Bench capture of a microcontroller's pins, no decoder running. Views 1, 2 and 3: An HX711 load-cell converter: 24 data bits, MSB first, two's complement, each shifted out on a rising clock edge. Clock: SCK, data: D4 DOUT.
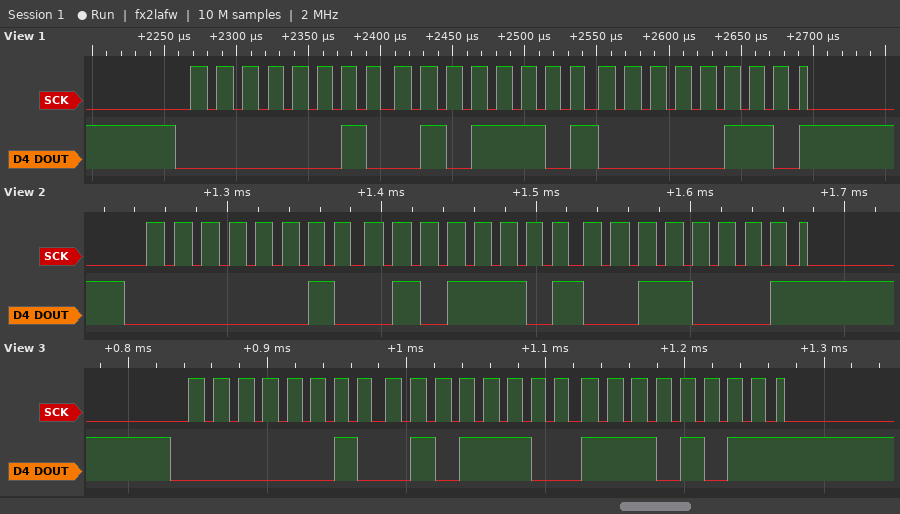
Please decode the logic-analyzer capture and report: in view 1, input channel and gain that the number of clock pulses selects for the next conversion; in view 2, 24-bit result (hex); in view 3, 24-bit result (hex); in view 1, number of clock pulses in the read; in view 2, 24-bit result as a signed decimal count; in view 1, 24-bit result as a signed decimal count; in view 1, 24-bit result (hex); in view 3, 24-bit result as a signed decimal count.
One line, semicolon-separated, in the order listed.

channel A, gain 128; 0x025D31; 0x025CEB; 25; 154929; 154886; 0x025D06; 154859
